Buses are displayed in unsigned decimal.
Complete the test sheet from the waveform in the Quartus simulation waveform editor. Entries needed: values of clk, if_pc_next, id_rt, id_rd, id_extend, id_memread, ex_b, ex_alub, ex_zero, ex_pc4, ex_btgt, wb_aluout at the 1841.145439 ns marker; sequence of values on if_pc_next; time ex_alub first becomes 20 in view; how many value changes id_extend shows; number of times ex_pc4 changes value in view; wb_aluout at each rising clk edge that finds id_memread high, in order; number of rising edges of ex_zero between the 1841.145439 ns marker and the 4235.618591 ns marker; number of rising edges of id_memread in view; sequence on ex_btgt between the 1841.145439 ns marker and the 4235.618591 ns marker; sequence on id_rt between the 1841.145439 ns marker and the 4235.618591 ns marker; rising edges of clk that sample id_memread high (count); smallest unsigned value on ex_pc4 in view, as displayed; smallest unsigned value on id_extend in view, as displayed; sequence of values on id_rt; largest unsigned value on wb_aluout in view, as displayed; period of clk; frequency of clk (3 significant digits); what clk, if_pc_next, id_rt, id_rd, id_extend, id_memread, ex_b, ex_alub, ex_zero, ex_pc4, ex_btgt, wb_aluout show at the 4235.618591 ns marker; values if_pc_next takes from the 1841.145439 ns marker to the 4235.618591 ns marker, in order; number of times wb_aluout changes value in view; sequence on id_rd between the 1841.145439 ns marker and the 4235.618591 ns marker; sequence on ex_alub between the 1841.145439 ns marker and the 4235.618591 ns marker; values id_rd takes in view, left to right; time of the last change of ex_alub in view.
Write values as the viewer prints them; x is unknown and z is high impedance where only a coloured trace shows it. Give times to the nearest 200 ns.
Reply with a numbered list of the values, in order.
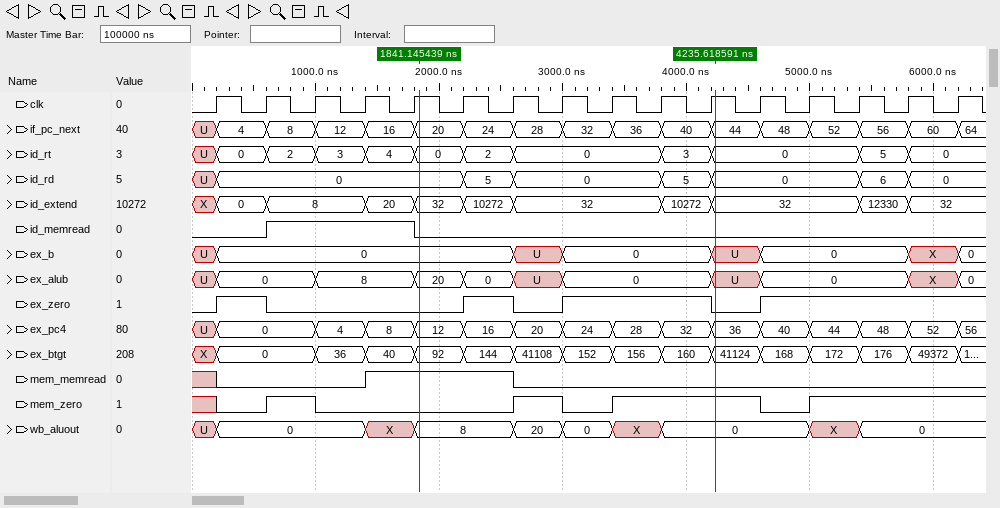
1. clk=1, if_pc_next=20, id_rt=0, id_rd=0, id_extend=32, id_memread=0, ex_b=0, ex_alub=20, ex_zero=0, ex_pc4=12, ex_btgt=92, wb_aluout=8
2. U, 4, 8, 12, 16, 20, 24, 28, 32, 36, 40, 44, 48, 52, 56, 60, 64
3. 1800 ns
4. 10
5. 15
6. 0, 0, X
7. 2
8. 1
9. 92, 144, 41108, 152, 156, 160, 41124
10. 0, 2, 0, 3, 0
11. 3
12. 0
13. 0
14. U, 0, 2, 3, 4, 0, 2, 0, 3, 0, 5, 0
15. 20
16. 400 ns
17. 2.50 MHz
18. clk=1, if_pc_next=44, id_rt=0, id_rd=0, id_extend=32, id_memread=0, ex_b=U, ex_alub=U, ex_zero=0, ex_pc4=36, ex_btgt=41124, wb_aluout=0
19. 20, 24, 28, 32, 36, 40, 44
20. 9
21. 0, 5, 0, 5, 0
22. 20, 0, U, 0, U
23. U, 0, 5, 0, 5, 0, 6, 0
24. 6200 ns
